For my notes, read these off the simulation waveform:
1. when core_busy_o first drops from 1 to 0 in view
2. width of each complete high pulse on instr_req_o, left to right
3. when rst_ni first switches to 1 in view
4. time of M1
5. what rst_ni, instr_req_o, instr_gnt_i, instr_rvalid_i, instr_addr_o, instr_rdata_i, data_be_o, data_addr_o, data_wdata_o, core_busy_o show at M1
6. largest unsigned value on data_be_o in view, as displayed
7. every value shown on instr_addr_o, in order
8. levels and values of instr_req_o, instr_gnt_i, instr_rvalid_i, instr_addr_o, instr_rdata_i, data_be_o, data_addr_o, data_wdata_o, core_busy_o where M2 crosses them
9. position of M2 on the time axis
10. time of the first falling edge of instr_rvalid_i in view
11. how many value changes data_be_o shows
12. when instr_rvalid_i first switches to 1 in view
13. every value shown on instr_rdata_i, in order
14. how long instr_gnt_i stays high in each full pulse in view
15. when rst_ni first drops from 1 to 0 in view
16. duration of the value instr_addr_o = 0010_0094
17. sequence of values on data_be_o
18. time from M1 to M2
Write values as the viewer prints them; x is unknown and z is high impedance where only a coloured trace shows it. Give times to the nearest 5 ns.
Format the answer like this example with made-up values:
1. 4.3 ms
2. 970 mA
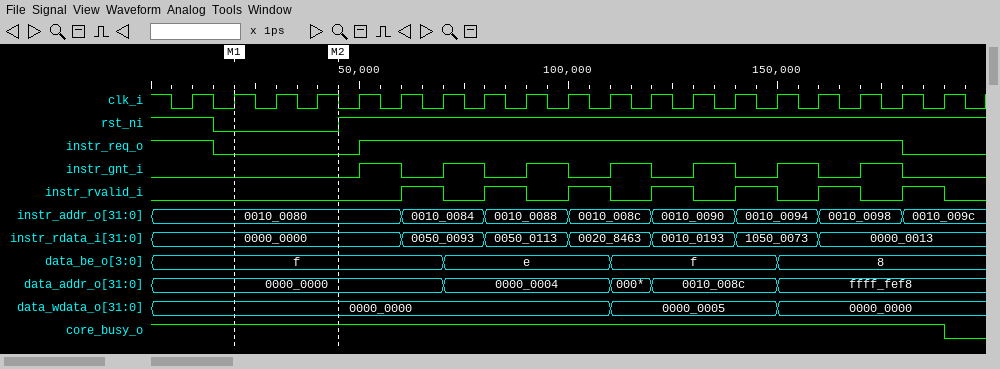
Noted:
1. 190 ns
2. 130 ns
3. 45 ns
4. 20 ns
5. rst_ni=0, instr_req_o=0, instr_gnt_i=0, instr_rvalid_i=0, instr_addr_o=0010_0080, instr_rdata_i=0000_0000, data_be_o=f, data_addr_o=0000_0000, data_wdata_o=0000_0000, core_busy_o=1
6. f
7. 0010_0080, 0010_0084, 0010_0088, 0010_008c, 0010_0090, 0010_0094, 0010_0098, 0010_009c
8. instr_req_o=0, instr_gnt_i=0, instr_rvalid_i=0, instr_addr_o=0010_0080, instr_rdata_i=0000_0000, data_be_o=f, data_addr_o=0000_0000, data_wdata_o=0000_0000, core_busy_o=1
9. 45 ns
10. 70 ns
11. 3
12. 60 ns
13. 0000_0000, 0050_0093, 0050_0113, 0020_8463, 0010_0193, 1050_0073, 0000_0013
14. 10 ns, 10 ns, 10 ns, 10 ns, 10 ns, 10 ns, 10 ns
15. 15 ns
16. 20 ns
17. f, e, f, 8
18. 25 ns
